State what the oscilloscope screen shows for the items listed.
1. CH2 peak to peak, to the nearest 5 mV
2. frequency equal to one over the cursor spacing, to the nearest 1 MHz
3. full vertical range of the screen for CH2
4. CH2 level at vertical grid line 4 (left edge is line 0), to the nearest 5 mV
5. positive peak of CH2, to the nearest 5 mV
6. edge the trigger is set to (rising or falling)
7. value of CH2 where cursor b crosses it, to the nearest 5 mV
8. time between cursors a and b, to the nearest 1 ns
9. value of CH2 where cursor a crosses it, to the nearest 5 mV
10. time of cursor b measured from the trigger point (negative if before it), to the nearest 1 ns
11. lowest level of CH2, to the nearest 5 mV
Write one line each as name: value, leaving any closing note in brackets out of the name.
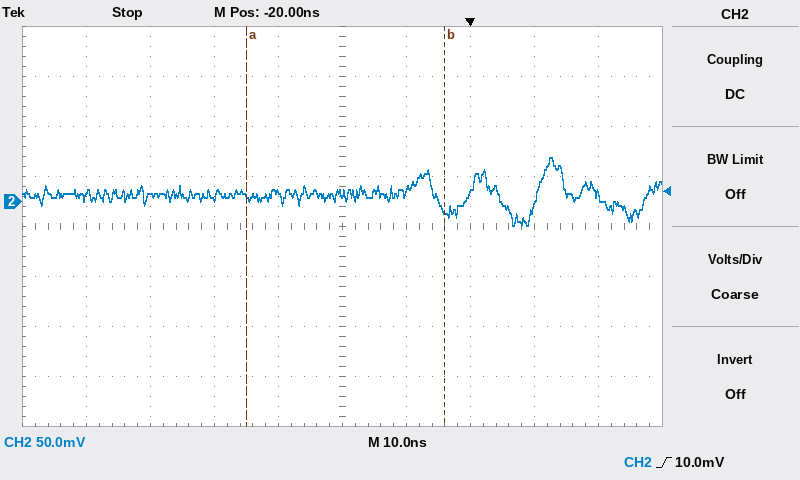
CH2 peak to peak, to the nearest 5 mV: 70 mV
frequency equal to one over the cursor spacing, to the nearest 1 MHz: 32 MHz
full vertical range of the screen for CH2: 400 mV
CH2 level at vertical grid line 4 (left edge is line 0), to the nearest 5 mV: 10 mV
positive peak of CH2, to the nearest 5 mV: 45 mV
edge the trigger is set to: rising
value of CH2 where cursor b crosses it, to the nearest 5 mV: -10 mV
time between cursors a and b, to the nearest 1 ns: 31 ns
value of CH2 where cursor a crosses it, to the nearest 5 mV: 5 mV
time of cursor b measured from the trigger point (negative if before it), to the nearest 1 ns: -4 ns
lowest level of CH2, to the nearest 5 mV: -25 mV
